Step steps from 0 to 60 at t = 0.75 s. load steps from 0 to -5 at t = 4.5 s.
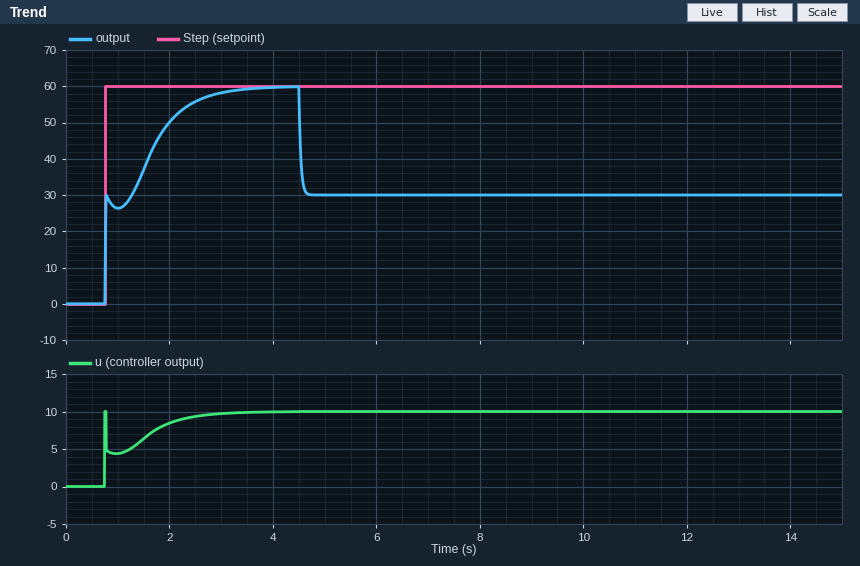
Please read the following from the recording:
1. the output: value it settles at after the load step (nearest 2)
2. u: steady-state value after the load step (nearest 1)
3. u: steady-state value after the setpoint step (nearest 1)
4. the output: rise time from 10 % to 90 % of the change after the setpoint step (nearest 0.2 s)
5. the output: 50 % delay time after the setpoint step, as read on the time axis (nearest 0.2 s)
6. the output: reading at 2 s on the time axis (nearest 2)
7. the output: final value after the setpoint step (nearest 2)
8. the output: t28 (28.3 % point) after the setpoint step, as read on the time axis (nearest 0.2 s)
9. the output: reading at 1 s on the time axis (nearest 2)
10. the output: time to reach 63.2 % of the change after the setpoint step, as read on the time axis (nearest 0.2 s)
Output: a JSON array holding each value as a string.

["30", "10", "10", "1.6 s", "1.2 s", "50", "60", "0.8 s", "26", "1.6 s"]
